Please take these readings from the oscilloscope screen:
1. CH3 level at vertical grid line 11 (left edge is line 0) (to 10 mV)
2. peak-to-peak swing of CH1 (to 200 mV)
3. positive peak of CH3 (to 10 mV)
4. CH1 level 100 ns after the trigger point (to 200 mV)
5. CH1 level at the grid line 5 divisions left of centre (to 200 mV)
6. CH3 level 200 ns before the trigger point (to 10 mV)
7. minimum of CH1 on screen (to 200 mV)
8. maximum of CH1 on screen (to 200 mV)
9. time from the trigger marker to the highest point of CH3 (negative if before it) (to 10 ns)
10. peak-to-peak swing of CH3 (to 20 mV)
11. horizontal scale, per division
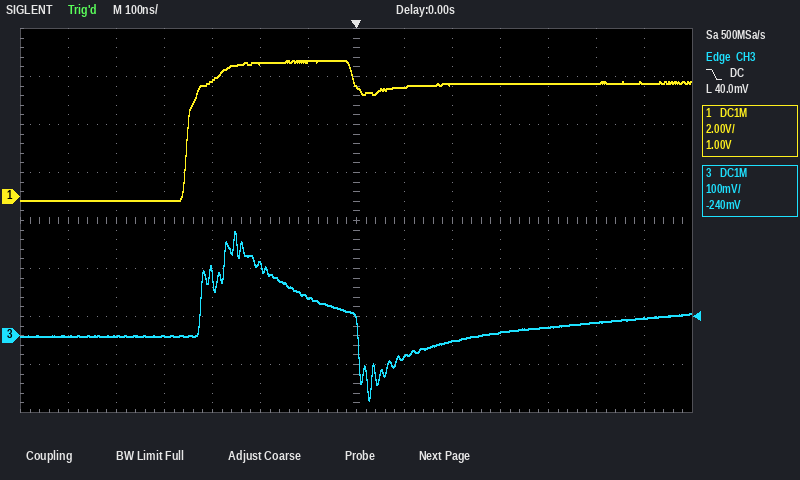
20 mV
5.8 V
220 mV
4.6 V
-200 mV
150 mV
-200 mV
5.6 V
-250 ns
360 mV
100 ns
